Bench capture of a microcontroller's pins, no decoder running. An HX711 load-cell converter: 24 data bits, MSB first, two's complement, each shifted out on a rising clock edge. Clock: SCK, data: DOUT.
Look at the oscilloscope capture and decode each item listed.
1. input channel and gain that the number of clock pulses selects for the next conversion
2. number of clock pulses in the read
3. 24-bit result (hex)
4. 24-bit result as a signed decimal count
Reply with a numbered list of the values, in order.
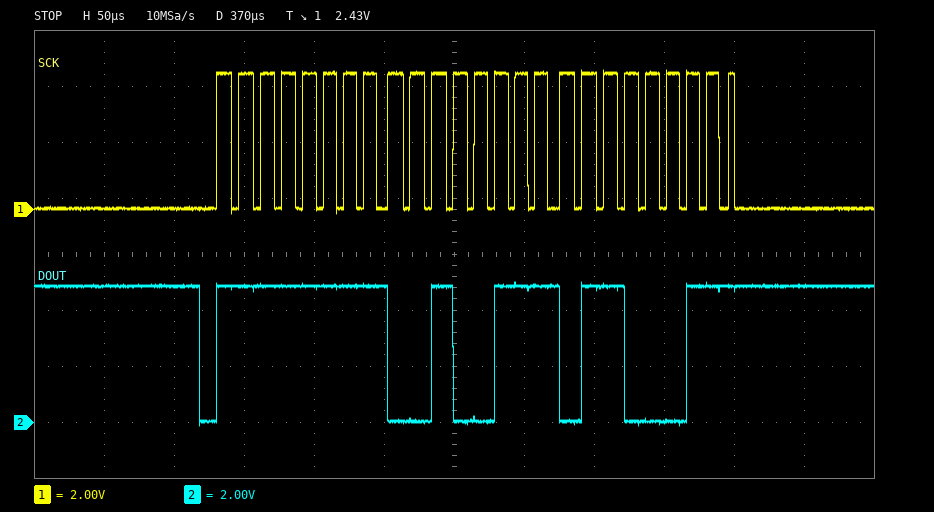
1. channel A, gain 128
2. 25
3. 0xFF2763
4. -55453
